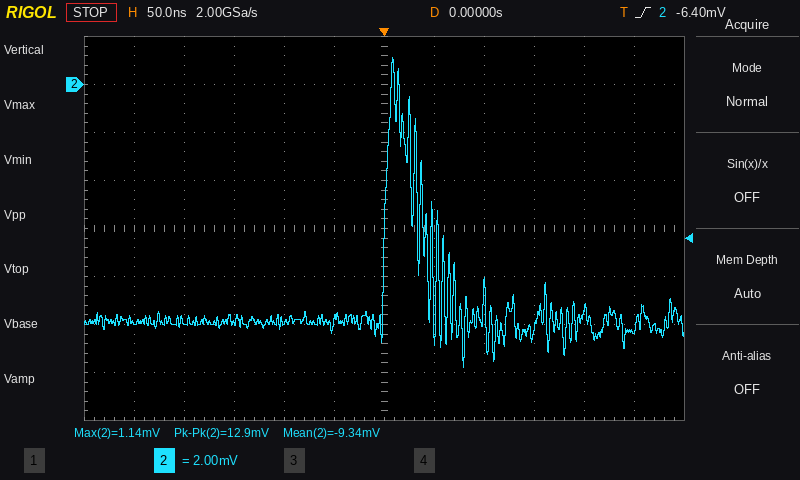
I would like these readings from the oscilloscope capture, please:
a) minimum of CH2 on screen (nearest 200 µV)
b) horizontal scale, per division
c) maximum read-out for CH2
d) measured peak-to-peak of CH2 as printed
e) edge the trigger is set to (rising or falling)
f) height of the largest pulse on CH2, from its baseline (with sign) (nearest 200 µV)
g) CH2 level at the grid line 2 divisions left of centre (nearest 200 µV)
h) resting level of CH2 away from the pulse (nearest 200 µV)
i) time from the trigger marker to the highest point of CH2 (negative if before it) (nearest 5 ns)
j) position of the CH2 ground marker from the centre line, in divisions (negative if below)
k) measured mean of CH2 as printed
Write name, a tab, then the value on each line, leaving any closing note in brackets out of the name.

minimum of CH2 on screen	-11.8 mV
horizontal scale, per division	50 ns
maximum read-out for CH2	1.14 mV
measured peak-to-peak of CH2 as printed	12.9 mV
edge the trigger is set to	rising
height of the largest pulse on CH2, from its baseline (with sign)	+11.0 mV
CH2 level at the grid line 2 divisions left of centre	-9.8 mV
resting level of CH2 away from the pulse	-9.8 mV
time from the trigger marker to the highest point of CH2 (negative if before it)	+10 ns
position of the CH2 ground marker from the centre line, in divisions	+3.0 div
measured mean of CH2 as printed	-9.34 mV
